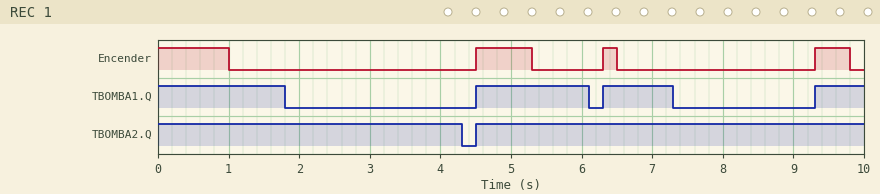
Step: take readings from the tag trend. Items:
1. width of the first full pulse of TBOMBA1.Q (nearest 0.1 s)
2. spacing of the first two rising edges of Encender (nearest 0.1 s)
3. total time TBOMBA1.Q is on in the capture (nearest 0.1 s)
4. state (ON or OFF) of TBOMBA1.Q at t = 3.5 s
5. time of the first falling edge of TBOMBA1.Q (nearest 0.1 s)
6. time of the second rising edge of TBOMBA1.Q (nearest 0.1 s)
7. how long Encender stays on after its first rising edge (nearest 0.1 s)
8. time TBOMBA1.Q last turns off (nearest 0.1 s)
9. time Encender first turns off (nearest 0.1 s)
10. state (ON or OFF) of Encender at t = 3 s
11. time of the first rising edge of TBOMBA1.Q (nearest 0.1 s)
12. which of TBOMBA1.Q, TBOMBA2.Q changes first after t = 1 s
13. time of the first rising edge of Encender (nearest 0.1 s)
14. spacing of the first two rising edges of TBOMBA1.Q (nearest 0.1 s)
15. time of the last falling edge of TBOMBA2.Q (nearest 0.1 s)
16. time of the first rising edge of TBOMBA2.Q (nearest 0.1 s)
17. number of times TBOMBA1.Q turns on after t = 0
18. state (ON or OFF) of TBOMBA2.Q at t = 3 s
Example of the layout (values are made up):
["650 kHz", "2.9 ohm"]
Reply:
["1.6 s", "1.8 s", "5.1 s", "OFF", "1.8 s", "6.3 s", "0.8 s", "7.3 s", "1.0 s", "OFF", "4.5 s", "TBOMBA1.Q", "4.5 s", "1.8 s", "4.3 s", "4.5 s", "3", "ON"]
